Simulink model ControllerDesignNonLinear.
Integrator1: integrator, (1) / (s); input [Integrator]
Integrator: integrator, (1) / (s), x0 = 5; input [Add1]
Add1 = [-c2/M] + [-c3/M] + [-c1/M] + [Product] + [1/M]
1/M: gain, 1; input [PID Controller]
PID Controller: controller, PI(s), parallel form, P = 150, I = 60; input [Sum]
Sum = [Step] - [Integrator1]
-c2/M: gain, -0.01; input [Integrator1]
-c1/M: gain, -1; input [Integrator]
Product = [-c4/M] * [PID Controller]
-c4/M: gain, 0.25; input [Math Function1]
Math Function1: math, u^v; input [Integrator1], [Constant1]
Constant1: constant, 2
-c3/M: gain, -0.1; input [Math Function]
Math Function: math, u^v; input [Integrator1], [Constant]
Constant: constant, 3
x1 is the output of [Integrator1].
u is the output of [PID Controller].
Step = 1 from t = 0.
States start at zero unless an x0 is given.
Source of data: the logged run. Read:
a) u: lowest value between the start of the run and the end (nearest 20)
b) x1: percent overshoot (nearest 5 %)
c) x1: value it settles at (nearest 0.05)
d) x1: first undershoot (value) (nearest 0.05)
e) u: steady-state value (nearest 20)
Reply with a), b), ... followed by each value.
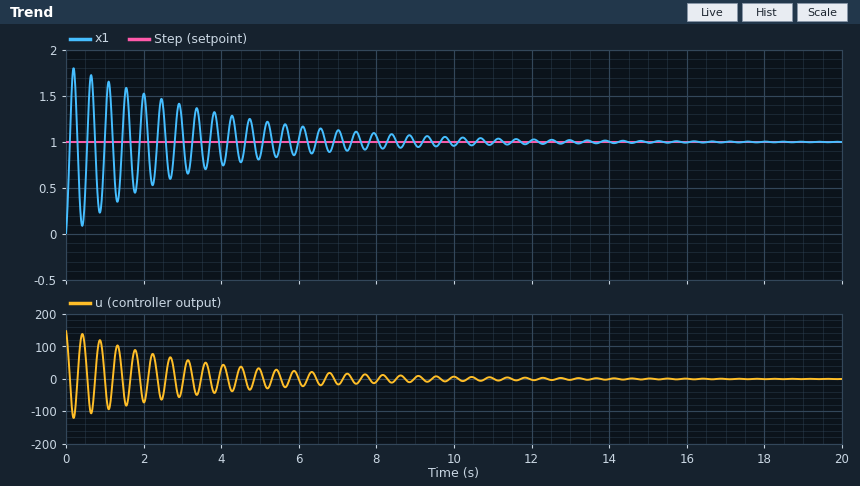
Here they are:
a) -120
b) 80 %
c) 1.00
d) 0.10
e) 0
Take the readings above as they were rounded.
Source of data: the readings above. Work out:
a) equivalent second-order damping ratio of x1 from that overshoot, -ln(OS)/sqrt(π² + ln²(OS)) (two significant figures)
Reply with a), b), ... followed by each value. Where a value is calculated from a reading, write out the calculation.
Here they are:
a) ln(0.8) = -0.223; 0.223 / sqrt(9.870 + 0.050) = 0.071
